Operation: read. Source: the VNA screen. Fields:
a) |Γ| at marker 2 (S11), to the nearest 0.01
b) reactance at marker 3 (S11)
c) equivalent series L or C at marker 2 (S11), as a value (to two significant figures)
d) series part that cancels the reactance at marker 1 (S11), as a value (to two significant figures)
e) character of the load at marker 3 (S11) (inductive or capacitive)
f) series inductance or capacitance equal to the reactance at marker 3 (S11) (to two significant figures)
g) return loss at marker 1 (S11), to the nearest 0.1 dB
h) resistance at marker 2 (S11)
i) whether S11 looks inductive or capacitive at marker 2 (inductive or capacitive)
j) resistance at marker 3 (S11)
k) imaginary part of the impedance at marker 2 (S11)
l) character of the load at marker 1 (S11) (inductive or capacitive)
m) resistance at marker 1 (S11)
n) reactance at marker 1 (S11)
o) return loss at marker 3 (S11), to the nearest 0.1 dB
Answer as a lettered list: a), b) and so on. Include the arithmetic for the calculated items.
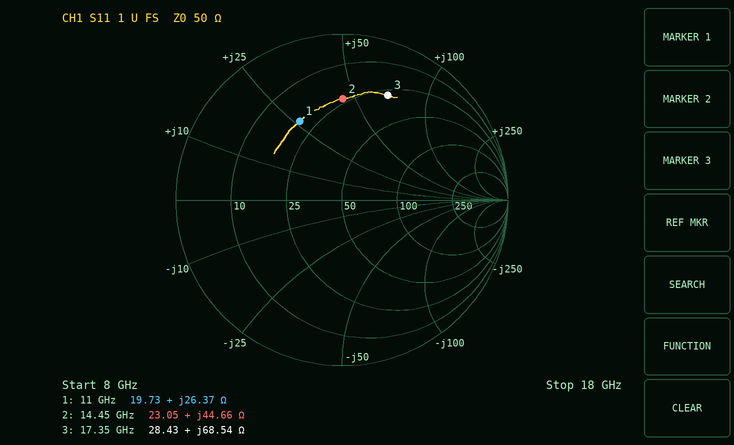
a) 0.61
b) +68.54 Ω
c) L = 44.66 Ω/(2π × 14.45 GHz) ≈ 492 pH, so 490 pH to two significant figures
d) C = 1/(2π × 11 GHz × 26.37 Ω) ≈ 549 fF, so 550 fF to two significant figures
e) inductive
f) L = 68.54 Ω/(2π × 17.35 GHz) ≈ 629 pH, so 630 pH to two significant figures
g) 5.4 dB
h) 23.05 Ω
i) inductive
j) 28.43 Ω
k) +44.66 Ω
l) inductive
m) 19.73 Ω
n) +26.37 Ω
o) 3.2 dB
